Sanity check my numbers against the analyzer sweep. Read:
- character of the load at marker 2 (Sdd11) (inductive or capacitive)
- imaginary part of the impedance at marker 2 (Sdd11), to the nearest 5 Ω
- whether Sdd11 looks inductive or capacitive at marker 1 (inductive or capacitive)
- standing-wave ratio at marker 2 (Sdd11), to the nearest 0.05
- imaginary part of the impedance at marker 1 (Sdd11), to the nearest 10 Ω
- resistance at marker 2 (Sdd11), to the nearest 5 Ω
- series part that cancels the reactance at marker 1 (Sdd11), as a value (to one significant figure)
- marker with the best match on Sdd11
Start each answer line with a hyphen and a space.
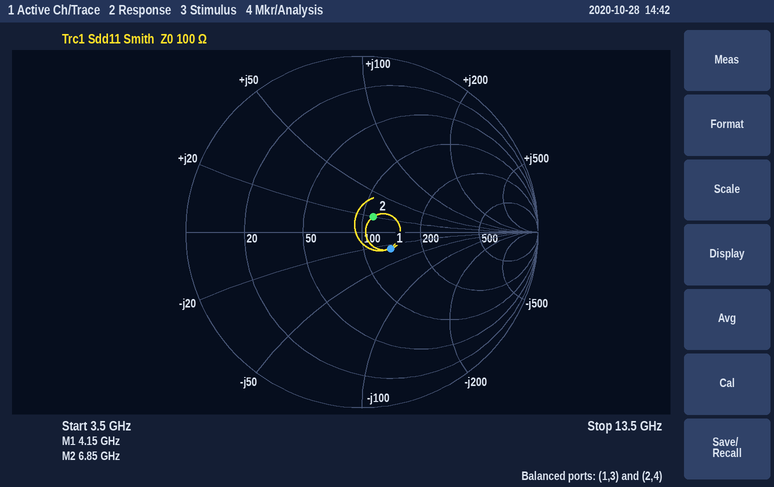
- inductive
- +20 Ω
- capacitive
- 1.25
- -30 Ω
- 110 Ω
- 1 nH
- marker 2
